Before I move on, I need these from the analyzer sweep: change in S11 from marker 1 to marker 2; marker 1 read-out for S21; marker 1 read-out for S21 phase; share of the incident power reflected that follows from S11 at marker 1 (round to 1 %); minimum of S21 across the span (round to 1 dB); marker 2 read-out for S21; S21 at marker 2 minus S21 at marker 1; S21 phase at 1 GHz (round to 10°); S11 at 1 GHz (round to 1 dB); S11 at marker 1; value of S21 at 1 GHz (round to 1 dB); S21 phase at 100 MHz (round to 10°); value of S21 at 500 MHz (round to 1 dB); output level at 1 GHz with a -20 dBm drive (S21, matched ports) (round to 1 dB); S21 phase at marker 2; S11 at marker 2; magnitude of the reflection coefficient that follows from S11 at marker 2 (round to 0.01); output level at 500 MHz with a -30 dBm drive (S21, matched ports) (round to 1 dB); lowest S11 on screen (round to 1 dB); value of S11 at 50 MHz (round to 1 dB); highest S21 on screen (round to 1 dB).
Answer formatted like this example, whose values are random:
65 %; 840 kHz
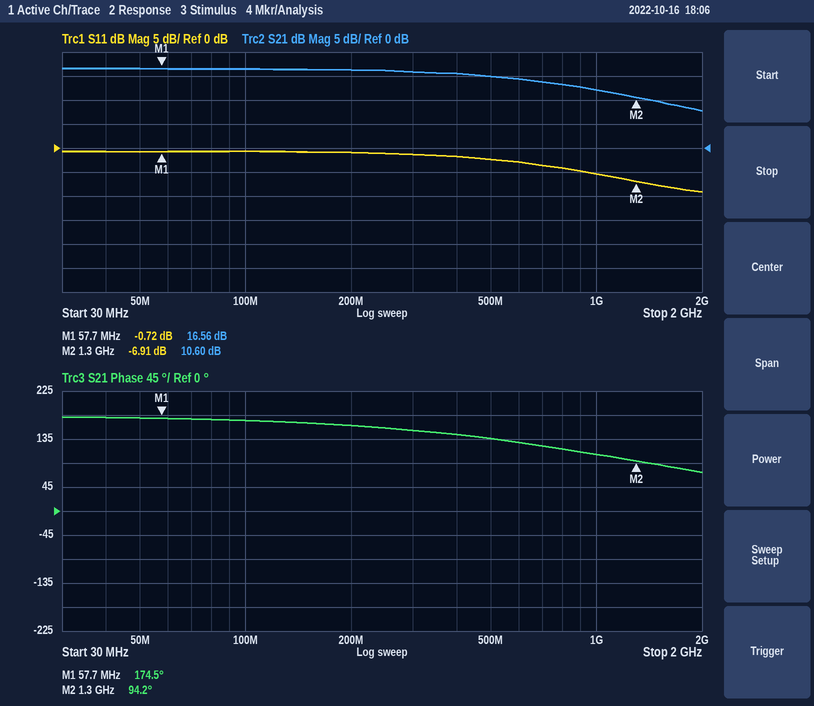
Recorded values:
-6.19 dB; 16.56 dB; 174.5°; 85 %; 8 dB; 10.60 dB; -5.96 dB; 110°; -5 dB; -0.72 dB; 12 dB; 170°; 15 dB; -8 dBm; 94.2°; -6.91 dB; 0.45; -15 dBm; -9 dB; -1 dB; 17 dB
